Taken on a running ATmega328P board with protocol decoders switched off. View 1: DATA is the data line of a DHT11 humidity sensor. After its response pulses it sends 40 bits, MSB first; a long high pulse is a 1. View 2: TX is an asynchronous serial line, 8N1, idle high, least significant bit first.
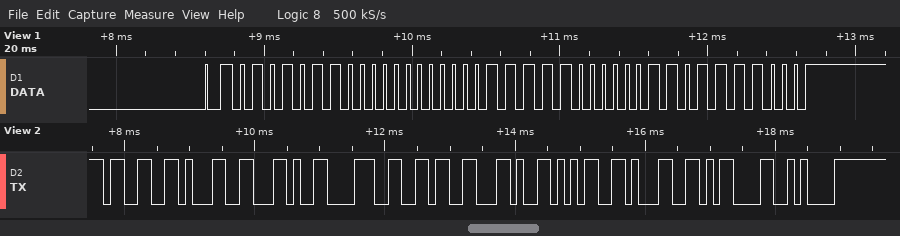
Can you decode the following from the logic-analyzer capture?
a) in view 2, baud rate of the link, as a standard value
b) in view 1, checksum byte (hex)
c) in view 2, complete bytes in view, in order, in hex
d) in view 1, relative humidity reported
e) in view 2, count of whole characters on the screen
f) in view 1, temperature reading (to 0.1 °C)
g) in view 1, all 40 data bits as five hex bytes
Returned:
9600 baud
0x78
33 31 2C 38 36 2C 35 31 0D 0A
86 %
10
31.3 °C
56 00 1F 03 78
